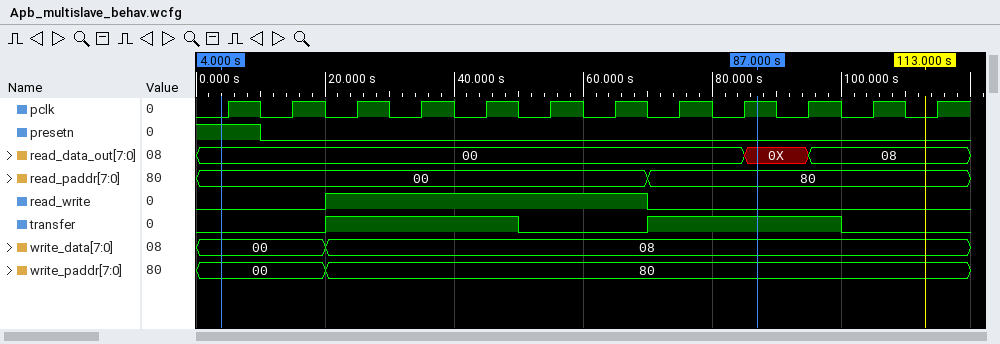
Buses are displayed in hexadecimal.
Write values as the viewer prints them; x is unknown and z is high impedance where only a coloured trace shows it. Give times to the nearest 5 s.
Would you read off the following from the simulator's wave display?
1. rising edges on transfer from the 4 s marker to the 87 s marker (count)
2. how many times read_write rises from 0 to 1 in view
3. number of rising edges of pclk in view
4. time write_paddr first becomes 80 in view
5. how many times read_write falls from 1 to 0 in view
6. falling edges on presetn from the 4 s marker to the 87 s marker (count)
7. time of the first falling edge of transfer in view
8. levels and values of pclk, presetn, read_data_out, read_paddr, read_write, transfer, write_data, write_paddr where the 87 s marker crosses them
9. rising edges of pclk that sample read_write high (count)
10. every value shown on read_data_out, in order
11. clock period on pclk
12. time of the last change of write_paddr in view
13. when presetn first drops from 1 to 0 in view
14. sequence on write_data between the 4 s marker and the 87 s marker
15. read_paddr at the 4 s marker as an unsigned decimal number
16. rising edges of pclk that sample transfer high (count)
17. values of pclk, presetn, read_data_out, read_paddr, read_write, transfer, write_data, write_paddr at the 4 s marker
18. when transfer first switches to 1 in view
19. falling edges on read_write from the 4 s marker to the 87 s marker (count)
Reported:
2
1
12
20 s
1
1
50 s
pclk=1, presetn=0, read_data_out=0X, read_paddr=80, read_write=0, transfer=1, write_data=08, write_paddr=80
5
00, 0X, 08
10 s
20 s
10 s
00, 08
0
6
pclk=0, presetn=1, read_data_out=00, read_paddr=00, read_write=0, transfer=0, write_data=00, write_paddr=00
20 s
1
